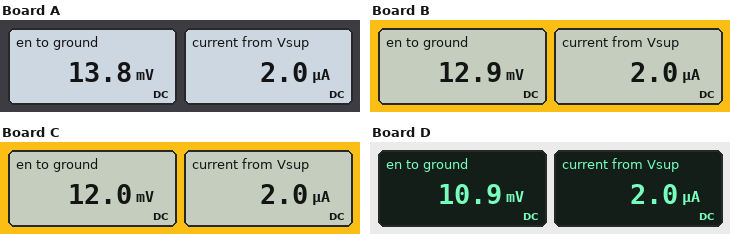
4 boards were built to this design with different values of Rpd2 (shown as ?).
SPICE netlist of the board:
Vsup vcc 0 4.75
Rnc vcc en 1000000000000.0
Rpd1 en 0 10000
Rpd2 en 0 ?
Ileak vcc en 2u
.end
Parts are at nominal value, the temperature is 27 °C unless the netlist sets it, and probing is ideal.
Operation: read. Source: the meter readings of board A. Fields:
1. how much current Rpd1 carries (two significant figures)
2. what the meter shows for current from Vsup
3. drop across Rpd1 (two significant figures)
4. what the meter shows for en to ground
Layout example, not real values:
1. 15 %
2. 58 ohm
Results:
1. 1.4 µA
2. 2.0 µA
3. 14 mV
4. 13.8 mV
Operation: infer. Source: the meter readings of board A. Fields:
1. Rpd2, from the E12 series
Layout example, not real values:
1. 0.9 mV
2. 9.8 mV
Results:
1. 22 kΩ
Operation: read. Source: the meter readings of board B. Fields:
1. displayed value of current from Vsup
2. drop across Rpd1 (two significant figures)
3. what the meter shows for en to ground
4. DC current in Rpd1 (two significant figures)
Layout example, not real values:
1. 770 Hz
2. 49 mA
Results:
1. 2.0 µA
2. 13 mV
3. 12.9 mV
4. 1.3 µA
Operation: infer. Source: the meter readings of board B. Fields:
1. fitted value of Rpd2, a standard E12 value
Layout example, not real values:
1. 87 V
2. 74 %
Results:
1. 18 kΩ
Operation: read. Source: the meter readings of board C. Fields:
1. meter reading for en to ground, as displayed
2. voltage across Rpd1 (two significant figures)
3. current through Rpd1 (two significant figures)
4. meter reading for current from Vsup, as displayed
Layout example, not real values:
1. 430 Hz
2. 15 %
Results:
1. 12.0 mV
2. 12 mV
3. 1.2 µA
4. 2.0 µA
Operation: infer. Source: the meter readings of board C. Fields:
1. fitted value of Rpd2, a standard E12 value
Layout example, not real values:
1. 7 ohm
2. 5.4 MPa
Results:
1. 15 kΩ
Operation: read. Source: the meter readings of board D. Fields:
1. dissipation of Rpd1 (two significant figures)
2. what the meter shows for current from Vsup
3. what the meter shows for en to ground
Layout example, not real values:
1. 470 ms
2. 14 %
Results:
1. 12 nW
2. 2.0 µA
3. 10.9 mV
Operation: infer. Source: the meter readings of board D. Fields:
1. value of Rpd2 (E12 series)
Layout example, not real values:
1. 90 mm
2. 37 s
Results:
1. 12 kΩ
